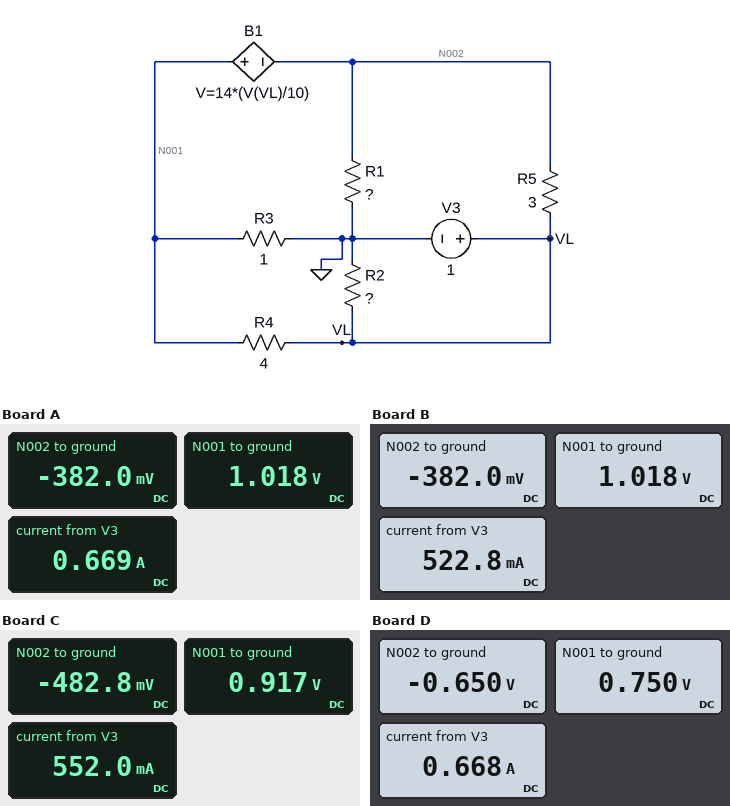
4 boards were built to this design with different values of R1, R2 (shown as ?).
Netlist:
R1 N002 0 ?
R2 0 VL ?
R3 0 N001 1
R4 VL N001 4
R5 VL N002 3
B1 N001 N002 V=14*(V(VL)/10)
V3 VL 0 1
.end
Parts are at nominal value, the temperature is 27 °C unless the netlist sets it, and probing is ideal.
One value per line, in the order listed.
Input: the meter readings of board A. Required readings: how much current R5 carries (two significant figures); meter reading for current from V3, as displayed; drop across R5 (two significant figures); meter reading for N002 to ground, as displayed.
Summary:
460 mA
0.669 A
1.4 V
-382.0 mV
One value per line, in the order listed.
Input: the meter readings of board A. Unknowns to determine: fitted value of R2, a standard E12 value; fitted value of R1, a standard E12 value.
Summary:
4.7 Ω
0.68 Ω
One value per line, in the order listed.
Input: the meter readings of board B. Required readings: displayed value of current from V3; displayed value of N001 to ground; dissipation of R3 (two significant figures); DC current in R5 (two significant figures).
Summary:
522.8 mA
1.018 V
1.0 W
460 mA
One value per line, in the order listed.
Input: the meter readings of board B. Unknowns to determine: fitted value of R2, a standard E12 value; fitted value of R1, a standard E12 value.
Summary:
15 Ω
0.68 Ω
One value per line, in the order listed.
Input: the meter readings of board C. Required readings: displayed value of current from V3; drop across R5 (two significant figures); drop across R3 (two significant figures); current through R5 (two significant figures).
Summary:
552.0 mA
1.5 V
920 mV
490 mA
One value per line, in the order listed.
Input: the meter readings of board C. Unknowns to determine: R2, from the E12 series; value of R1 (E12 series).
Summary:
27 Ω
1.2 Ω
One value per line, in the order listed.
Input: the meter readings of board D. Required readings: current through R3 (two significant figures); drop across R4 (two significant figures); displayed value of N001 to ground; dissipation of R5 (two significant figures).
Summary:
750 mA
250 mV
0.750 V
910 mW
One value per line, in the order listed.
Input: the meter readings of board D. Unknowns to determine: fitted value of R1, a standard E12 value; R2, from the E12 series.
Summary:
4.7 Ω
18 Ω
